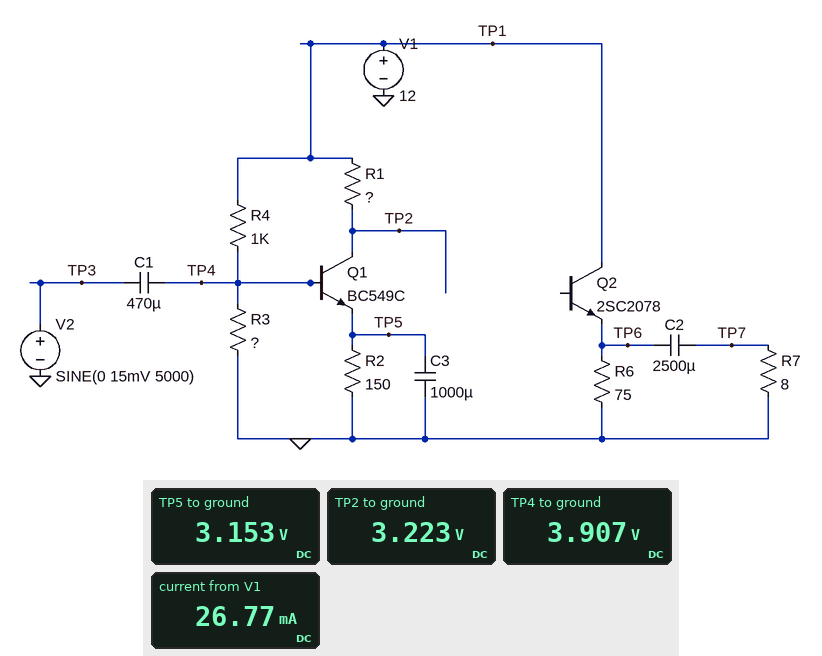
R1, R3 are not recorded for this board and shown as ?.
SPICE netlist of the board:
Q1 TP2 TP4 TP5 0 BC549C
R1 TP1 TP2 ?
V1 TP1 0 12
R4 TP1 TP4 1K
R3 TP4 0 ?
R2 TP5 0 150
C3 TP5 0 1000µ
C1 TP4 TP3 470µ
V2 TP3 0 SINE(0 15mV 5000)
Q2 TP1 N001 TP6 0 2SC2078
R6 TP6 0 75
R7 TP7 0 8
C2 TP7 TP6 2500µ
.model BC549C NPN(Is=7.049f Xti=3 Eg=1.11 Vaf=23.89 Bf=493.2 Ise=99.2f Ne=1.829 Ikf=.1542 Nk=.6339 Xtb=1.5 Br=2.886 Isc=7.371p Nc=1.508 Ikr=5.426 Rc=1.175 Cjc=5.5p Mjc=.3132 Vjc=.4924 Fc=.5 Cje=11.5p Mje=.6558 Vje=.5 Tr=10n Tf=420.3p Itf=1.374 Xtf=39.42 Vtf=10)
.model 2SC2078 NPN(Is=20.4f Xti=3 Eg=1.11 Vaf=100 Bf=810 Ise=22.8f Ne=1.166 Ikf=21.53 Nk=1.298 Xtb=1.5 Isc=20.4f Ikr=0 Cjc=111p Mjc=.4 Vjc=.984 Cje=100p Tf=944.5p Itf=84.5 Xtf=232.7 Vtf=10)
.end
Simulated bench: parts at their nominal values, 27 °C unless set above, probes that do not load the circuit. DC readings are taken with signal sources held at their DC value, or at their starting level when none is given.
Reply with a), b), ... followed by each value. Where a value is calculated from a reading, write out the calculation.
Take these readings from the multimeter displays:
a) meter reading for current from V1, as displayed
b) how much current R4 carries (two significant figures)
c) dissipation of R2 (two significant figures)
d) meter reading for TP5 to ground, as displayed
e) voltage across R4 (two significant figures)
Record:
a) 26.77 mA
b) (12 V - 3.907 V) / 1 kΩ = 8.1 mA
c) (3.153 V)^2 / 150 Ω = 66 mW
d) 3.153 V
e) 12 V - 3.907 V = 8.1 V
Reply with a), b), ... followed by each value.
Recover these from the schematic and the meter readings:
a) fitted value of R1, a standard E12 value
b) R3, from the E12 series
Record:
a) 470 Ω
b) 680 Ω
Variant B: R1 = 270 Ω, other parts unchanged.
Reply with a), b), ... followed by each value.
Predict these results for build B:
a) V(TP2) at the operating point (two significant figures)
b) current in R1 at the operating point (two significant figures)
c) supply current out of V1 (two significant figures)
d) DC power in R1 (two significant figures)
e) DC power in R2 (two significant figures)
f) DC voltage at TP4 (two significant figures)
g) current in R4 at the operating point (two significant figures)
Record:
a) 4.7 V
b) 27 mA
c) 34 mA
d) 200 mW
e) 110 mW
f) 4.8 V
g) 7.2 mA
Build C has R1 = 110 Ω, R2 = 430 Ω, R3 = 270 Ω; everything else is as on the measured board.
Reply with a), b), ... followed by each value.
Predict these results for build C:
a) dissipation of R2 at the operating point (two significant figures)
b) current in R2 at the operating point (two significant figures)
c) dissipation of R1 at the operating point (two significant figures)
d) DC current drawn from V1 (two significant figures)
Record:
a) 8.0 mW
b) 4.3 mA
c) 2.0 mW
d) 14 mA
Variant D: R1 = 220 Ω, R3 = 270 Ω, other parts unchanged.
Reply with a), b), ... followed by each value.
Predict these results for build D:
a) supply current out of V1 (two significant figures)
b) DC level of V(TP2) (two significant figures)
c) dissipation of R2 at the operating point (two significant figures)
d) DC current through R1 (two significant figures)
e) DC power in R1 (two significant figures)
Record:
a) 22 mA
b) 9.3 V
c) 22 mW
d) 12 mA
e) 32 mW
